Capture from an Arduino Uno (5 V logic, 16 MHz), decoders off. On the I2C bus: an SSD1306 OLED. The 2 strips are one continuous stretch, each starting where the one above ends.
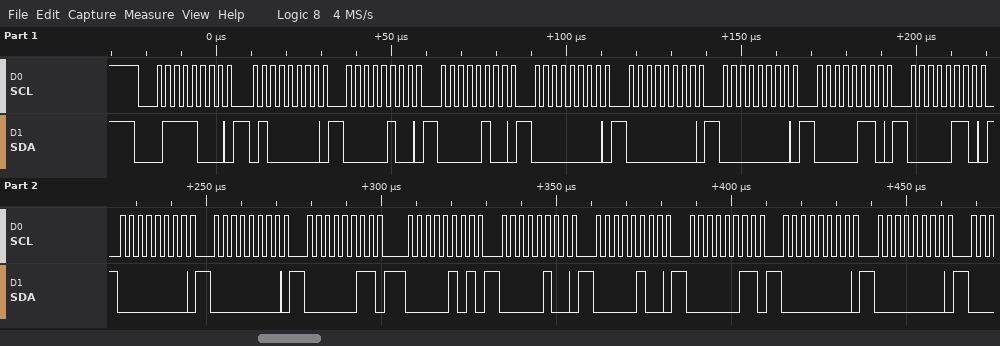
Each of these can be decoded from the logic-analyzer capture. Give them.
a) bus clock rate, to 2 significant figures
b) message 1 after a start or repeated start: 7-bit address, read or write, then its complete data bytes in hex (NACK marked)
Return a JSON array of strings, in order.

["400 kHz", "0x3C write: 40 04 04 00 00 00 06 06 00 00 03 05 04 04 03 00 00"]
